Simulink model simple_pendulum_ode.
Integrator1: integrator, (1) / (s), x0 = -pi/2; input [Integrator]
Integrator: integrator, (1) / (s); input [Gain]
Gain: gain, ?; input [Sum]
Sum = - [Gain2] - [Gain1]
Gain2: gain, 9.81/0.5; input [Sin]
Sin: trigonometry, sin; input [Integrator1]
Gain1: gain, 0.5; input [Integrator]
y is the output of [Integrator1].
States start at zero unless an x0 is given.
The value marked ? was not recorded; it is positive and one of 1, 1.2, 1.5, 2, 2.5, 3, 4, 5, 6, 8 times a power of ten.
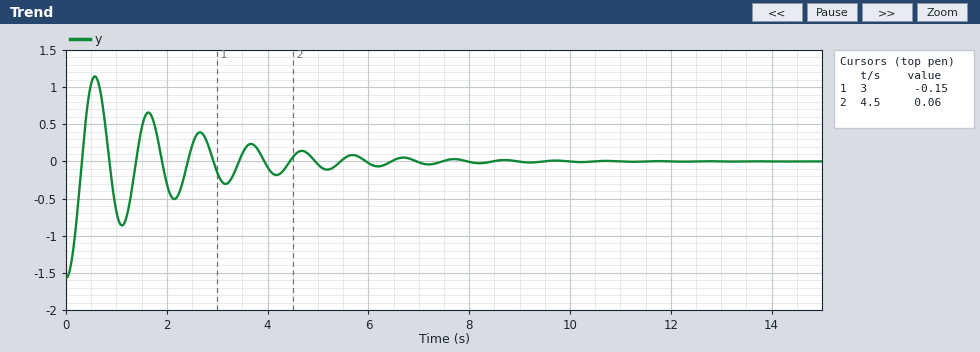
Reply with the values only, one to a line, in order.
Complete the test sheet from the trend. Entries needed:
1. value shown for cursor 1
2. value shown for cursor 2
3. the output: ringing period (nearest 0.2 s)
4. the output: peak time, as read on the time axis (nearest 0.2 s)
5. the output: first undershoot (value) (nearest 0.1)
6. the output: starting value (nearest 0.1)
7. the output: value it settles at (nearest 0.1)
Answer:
-0.15
0.06
1.0 s
0.6 s
-0.9
-1.6
0.0
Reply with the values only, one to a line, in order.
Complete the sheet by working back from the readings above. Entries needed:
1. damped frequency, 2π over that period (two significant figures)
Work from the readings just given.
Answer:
6.3 rad/s
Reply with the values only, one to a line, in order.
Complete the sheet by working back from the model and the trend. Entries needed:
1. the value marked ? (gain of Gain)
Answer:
2
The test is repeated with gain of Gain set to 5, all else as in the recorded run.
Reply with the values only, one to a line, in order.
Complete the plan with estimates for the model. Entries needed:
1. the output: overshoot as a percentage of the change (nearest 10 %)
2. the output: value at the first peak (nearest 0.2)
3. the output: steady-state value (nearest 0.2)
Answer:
60 %
1.0
0.0
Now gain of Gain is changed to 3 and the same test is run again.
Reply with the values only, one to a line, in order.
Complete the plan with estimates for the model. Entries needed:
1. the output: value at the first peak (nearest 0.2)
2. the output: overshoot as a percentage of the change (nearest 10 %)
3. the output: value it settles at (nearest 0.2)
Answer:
1.0
70 %
0.0
